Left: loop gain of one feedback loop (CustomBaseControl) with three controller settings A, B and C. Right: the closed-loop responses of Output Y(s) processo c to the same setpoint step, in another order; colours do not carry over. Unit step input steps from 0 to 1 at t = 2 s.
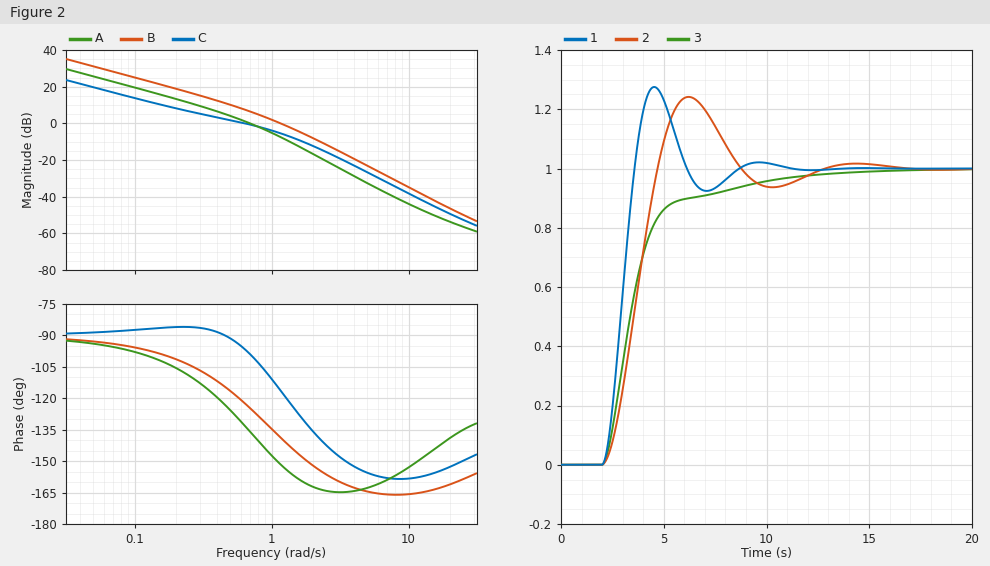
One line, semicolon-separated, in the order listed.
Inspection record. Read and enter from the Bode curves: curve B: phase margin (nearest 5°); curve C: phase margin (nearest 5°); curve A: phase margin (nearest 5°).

40°; 85°; 45°
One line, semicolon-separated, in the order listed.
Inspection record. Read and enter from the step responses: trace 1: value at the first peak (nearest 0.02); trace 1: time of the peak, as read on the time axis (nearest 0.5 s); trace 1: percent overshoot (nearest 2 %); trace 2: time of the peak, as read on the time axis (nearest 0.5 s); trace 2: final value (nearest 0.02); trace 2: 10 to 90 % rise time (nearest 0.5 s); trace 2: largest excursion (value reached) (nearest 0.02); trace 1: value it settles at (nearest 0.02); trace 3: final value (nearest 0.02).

1.28; 4.5 s; 28 %; 6.0 s; 1.00; 2.0 s; 1.24; 1.00; 1.00
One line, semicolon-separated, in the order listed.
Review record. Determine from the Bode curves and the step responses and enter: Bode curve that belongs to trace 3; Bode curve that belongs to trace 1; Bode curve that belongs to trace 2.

C; B; A
